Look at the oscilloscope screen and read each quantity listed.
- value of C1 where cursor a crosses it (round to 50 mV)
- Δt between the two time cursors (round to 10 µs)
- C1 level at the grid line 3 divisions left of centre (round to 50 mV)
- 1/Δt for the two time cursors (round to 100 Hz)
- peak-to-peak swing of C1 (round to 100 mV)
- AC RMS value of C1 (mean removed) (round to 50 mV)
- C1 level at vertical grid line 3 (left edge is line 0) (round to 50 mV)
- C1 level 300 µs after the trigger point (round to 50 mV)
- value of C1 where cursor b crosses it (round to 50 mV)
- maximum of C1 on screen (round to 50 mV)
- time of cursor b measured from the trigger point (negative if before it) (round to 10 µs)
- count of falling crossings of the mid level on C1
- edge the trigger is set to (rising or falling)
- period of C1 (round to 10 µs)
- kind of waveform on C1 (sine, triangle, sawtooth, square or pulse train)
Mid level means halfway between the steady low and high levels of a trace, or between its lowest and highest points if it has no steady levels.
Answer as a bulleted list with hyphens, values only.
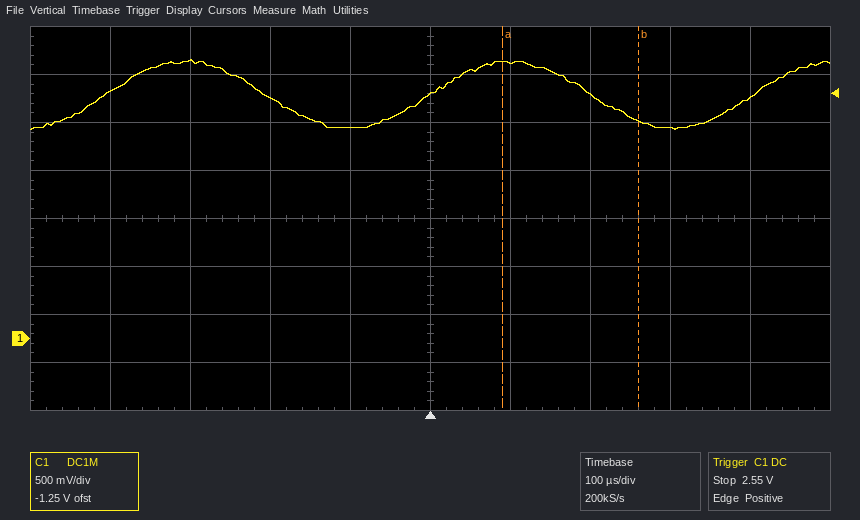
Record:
- 2.90 V
- 170 µs
- 2.90 V
- 5.9 kHz
- 700 mV
- 250 mV
- 2.50 V
- 2.20 V
- 2.25 V
- 2.90 V
- +260 µs
- 2
- rising
- 410 µs
- sine
